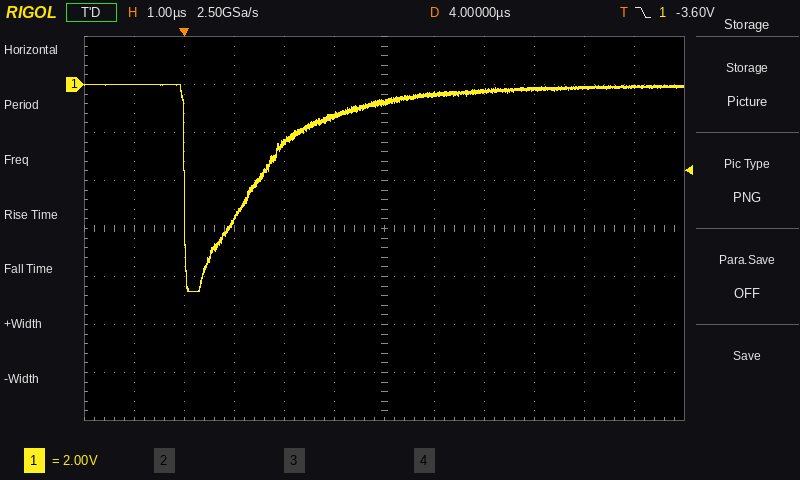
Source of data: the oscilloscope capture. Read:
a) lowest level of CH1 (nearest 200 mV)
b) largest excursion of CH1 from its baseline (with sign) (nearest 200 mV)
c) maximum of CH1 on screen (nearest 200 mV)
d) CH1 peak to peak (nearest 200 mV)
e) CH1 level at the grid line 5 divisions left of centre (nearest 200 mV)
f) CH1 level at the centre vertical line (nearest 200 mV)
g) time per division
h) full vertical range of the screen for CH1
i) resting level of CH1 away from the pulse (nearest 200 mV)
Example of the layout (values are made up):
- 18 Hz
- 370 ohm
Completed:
- -8.6 V
- -8.4 V
- 0.0 V
- 8.6 V
- 0.0 V
- -800 mV
- 1 µs
- 16 V
- -200 mV
